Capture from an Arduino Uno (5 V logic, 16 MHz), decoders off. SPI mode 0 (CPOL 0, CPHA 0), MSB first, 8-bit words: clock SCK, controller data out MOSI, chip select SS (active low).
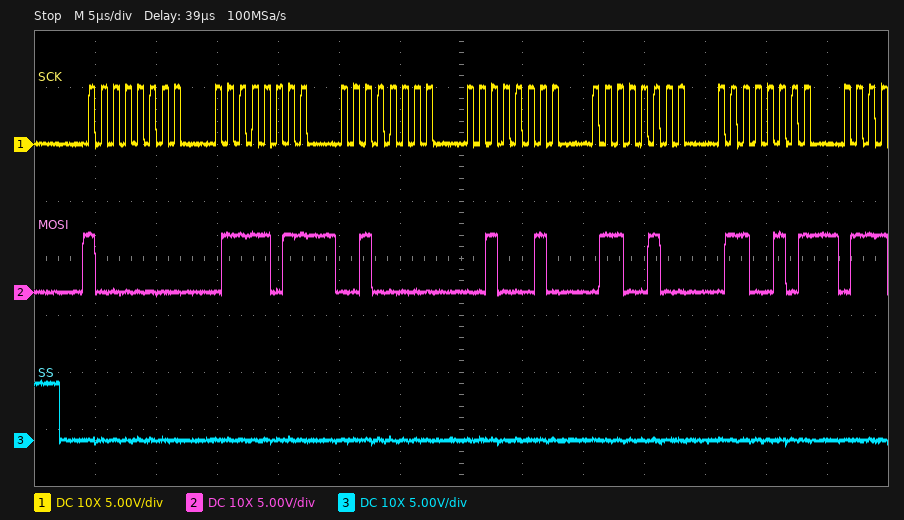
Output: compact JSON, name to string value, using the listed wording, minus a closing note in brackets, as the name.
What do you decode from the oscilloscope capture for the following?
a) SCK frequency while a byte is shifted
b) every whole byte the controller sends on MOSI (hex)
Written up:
{"SCK frequency while a byte is shifted": "1 MHz", "every whole byte the controller sends on MOSI": "80 7B 20 22 64 65"}
